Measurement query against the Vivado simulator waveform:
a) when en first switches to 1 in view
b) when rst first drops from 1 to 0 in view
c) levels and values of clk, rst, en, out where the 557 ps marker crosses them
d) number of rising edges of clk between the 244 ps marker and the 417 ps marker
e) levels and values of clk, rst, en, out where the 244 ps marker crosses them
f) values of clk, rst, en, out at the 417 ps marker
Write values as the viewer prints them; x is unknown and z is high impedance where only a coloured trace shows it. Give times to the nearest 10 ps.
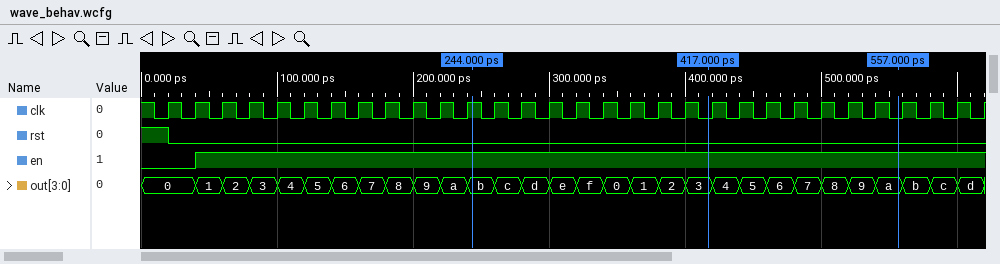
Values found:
40 ps
20 ps
clk=0, rst=0, en=1, out=a
8
clk=1, rst=0, en=1, out=b
clk=0, rst=0, en=1, out=3
